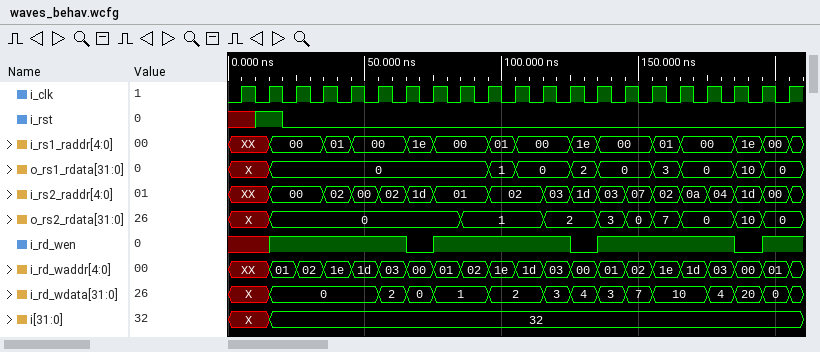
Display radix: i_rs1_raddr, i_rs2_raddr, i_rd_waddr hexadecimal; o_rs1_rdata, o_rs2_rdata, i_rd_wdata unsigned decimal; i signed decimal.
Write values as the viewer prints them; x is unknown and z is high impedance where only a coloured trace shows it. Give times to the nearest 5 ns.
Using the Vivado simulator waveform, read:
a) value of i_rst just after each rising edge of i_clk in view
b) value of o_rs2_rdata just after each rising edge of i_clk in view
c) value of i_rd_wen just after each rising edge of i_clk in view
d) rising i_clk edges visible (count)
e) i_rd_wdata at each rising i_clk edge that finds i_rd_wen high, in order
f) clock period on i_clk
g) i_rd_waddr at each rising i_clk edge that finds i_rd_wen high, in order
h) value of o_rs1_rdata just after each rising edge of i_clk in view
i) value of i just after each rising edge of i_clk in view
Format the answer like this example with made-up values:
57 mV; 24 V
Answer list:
x 1 0 0 0 0 0 0 0 0 0 0 0 0 0 0 0 0 0 0 0; X, 0, 0, 0, 0, 0, 0, 0, 1, 1, 1, 2, 2, 3, 0, 7, 0, 0, 10, 0, 0; x 1 1 1 1 1 0 1 1 1 1 1 0 1 1 1 1 1 0 1 1; 21; 0, 0, 0, 0, 2, 1, 1, 2, 2, 3, 3, 7, 10, 10, 4, 0; 10 ns; 01, 02, 1e, 1d, 03, 01, 02, 1e, 1d, 03, 01, 02, 1e, 1d, 03, 01; X, 0, 0, 0, 0, 0, 0, 0, 0, 1, 0, 0, 2, 0, 0, 3, 0, 0, 10, 0, 0; X, 32, 32, 32, 32, 32, 32, 32, 32, 32, 32, 32, 32, 32, 32, 32, 32, 32, 32, 32, 32
